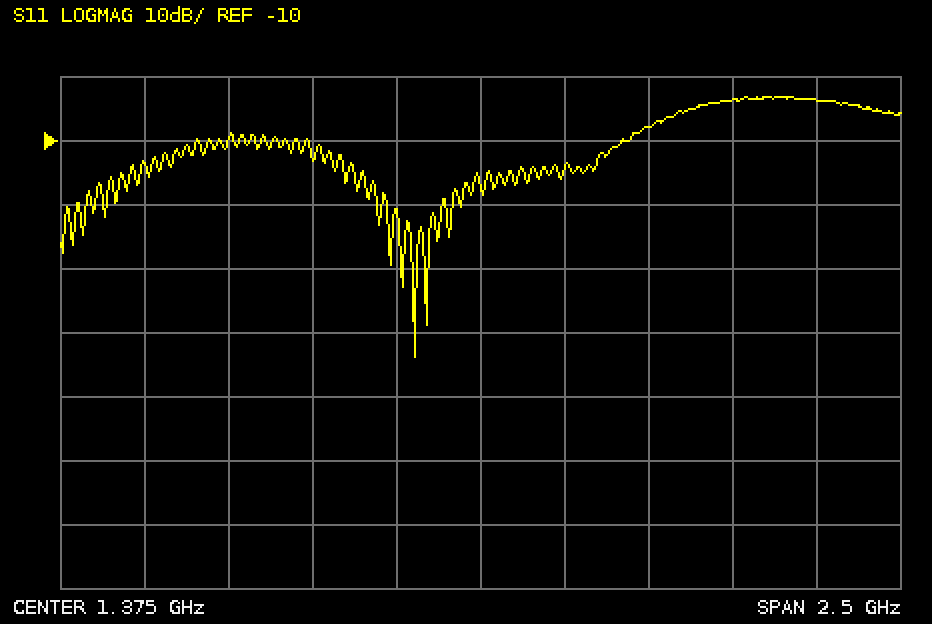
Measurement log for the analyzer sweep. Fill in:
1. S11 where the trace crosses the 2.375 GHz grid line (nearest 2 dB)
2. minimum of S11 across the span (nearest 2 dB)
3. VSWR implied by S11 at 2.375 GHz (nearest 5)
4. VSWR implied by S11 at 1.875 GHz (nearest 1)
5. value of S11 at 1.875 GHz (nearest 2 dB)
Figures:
-4 dB
-44 dB
5
2
-8 dB
